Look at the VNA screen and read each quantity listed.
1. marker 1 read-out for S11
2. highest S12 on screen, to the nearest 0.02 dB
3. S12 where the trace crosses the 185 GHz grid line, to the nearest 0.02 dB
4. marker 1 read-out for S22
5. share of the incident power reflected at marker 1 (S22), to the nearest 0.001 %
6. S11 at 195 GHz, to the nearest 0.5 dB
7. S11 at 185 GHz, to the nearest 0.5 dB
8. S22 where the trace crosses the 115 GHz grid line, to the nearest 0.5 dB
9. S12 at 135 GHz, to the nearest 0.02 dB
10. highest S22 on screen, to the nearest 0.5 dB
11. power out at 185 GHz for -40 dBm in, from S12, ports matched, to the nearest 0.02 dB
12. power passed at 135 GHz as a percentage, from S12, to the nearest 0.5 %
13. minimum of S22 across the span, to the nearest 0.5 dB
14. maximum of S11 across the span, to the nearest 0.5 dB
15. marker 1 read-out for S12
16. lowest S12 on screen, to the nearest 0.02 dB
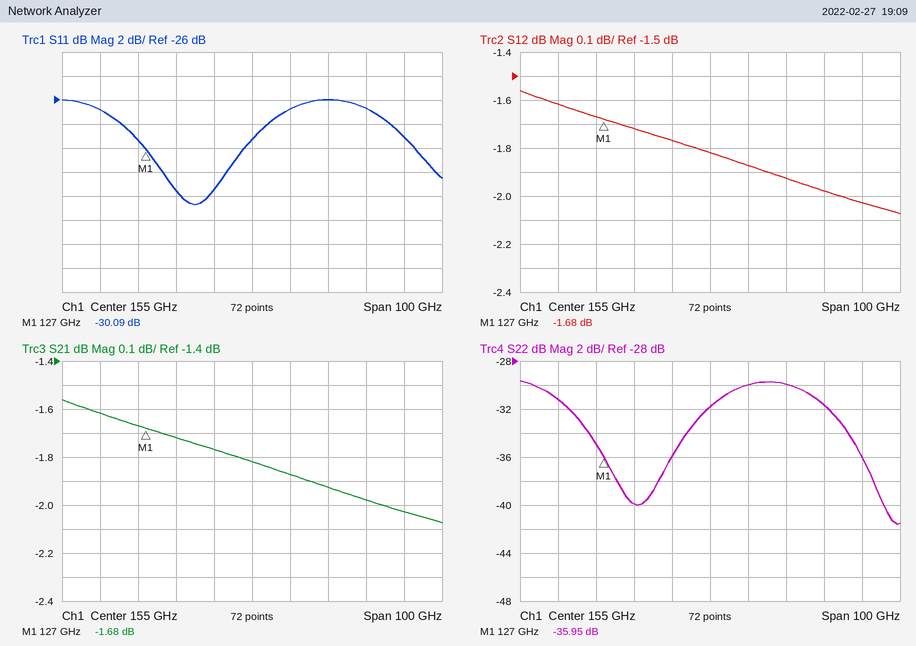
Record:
-30.09 dB
-1.56 dB
-1.98 dB
-35.95 dB
0.025 %
-29.0 dB
-26.5 dB
-31.0 dB
-1.72 dB
-29.5 dB
-41.98 dBm
67.5 %
-41.5 dB
-26.0 dB
-1.68 dB
-2.08 dB
